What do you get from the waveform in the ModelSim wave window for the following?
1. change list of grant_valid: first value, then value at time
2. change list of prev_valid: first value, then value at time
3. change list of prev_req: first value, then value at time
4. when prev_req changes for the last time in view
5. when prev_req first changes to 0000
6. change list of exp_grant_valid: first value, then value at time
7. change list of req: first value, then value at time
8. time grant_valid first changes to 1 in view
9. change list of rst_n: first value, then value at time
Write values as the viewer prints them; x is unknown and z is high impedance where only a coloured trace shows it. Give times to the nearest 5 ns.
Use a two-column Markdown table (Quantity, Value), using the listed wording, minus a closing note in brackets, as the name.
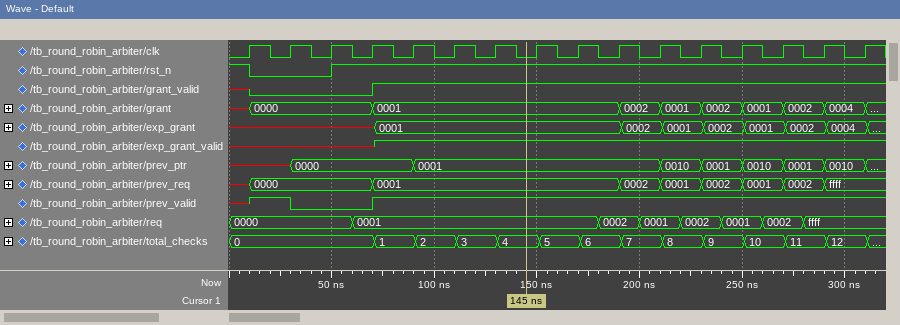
| Quantity | Value |
|---|---|
| change list of grant_valid: first value, then value at time | x, 0 at 10 ns, 1 at 70 ns |
| change list of prev_valid: first value, then value at time | x, 1 at 10 ns, 0 at 30 ns, 1 at 70 ns |
| change list of prev_req: first value, then value at time | x, 0000 at 10 ns, 0001 at 70 ns, 0002 at 190 ns, 0001 at 210 ns, 0002 at 230 ns, 0001 at 250 ns, 0002 at 270 ns, ffff at 290 ns |
| when prev_req changes for the last time in view | 290 ns |
| when prev_req first changes to 0000 | 10 ns |
| change list of exp_grant_valid: first value, then value at time | x, 1 at 70 ns |
| change list of req: first value, then value at time | 0000, 0001 at 60 ns, 0002 at 180 ns, 0001 at 200 ns, 0002 at 220 ns, 0001 at 240 ns, 0002 at 260 ns, ffff at 280 ns |
| time grant_valid first changes to 1 in view | 70 ns |
| change list of rst_n: first value, then value at time | 1, 0 at 10 ns, 1 at 50 ns |
